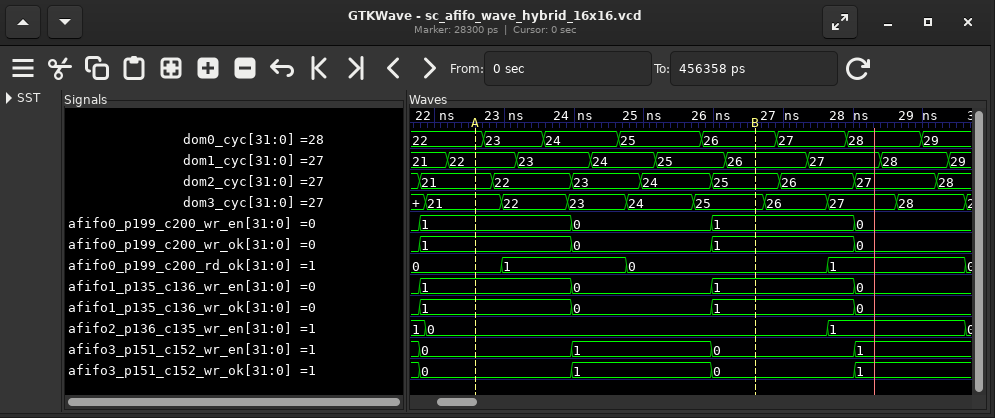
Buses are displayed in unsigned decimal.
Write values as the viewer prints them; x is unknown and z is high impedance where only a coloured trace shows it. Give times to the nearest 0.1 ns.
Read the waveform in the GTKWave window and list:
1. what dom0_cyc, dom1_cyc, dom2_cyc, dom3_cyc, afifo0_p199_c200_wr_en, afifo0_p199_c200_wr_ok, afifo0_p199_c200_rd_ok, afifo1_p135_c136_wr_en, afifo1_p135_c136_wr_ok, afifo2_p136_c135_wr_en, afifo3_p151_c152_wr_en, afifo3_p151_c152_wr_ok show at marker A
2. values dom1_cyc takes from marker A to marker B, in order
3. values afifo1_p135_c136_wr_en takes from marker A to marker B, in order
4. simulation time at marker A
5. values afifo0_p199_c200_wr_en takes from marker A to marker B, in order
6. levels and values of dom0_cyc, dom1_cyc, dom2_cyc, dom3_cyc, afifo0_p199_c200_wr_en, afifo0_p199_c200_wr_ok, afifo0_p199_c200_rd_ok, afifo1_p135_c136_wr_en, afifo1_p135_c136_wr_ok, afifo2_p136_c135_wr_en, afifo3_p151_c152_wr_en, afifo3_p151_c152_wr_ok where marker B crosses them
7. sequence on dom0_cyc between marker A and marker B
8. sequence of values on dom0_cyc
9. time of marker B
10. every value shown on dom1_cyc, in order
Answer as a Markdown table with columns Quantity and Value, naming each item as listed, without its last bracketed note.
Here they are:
| Quantity | Value |
|---|---|
| what dom0_cyc, dom1_cyc, dom2_cyc, dom3_cyc, afifo0_p199_c200_wr_en, afifo0_p199_c200_wr_ok, afifo0_p199_c200_rd_ok, afifo1_p135_c136_wr_en, afifo1_p135_c136_wr_ok, afifo2_p136_c135_wr_en, afifo3_p151_c152_wr_en, afifo3_p151_c152_wr_ok show at marker A | dom0_cyc=22, dom1_cyc=22, dom2_cyc=21, dom3_cyc=21, afifo0_p199_c200_wr_en=1, afifo0_p199_c200_wr_ok=1, afifo0_p199_c200_rd_ok=0, afifo1_p135_c136_wr_en=1, afifo1_p135_c136_wr_ok=1, afifo2_p136_c135_wr_en=0, afifo3_p151_c152_wr_en=0, afifo3_p151_c152_wr_ok=0 |
| values dom1_cyc takes from marker A to marker B, in order | 22, 23, 24, 25, 26 |
| values afifo1_p135_c136_wr_en takes from marker A to marker B, in order | 1, 0, 1 |
| simulation time at marker A | 22.6 ns |
| values afifo0_p199_c200_wr_en takes from marker A to marker B, in order | 1, 0, 1 |
| levels and values of dom0_cyc, dom1_cyc, dom2_cyc, dom3_cyc, afifo0_p199_c200_wr_en, afifo0_p199_c200_wr_ok, afifo0_p199_c200_rd_ok, afifo1_p135_c136_wr_en, afifo1_p135_c136_wr_ok, afifo2_p136_c135_wr_en, afifo3_p151_c152_wr_en, afifo3_p151_c152_wr_ok where marker B crosses them | dom0_cyc=26, dom1_cyc=26, dom2_cyc=25, dom3_cyc=25, afifo0_p199_c200_wr_en=1, afifo0_p199_c200_wr_ok=1, afifo0_p199_c200_rd_ok=0, afifo1_p135_c136_wr_en=1, afifo1_p135_c136_wr_ok=1, afifo2_p136_c135_wr_en=0, afifo3_p151_c152_wr_en=0, afifo3_p151_c152_wr_ok=0 |
| sequence on dom0_cyc between marker A and marker B | 22, 23, 24, 25, 26 |
| sequence of values on dom0_cyc | 22, 23, 24, 25, 26, 27, 28, 29 |
| time of marker B | 26.6 ns |
| every value shown on dom1_cyc, in order | 21, 22, 23, 24, 25, 26, 27, 28, 29 |
